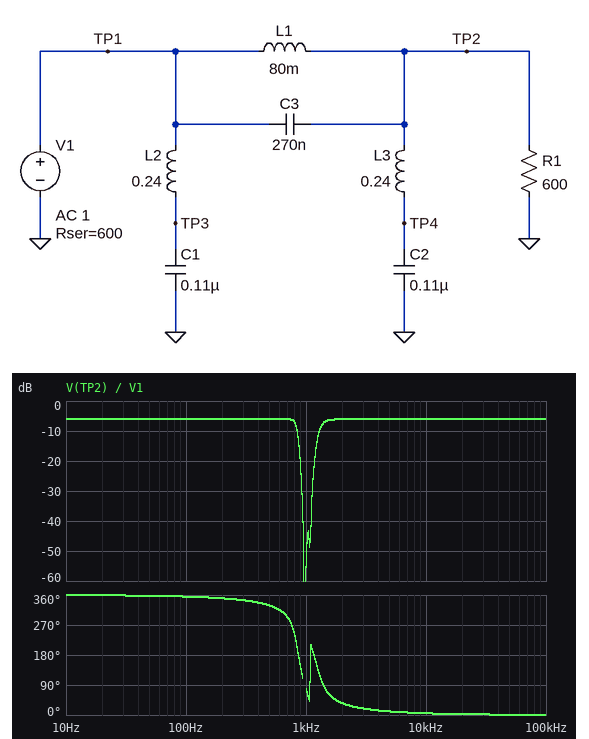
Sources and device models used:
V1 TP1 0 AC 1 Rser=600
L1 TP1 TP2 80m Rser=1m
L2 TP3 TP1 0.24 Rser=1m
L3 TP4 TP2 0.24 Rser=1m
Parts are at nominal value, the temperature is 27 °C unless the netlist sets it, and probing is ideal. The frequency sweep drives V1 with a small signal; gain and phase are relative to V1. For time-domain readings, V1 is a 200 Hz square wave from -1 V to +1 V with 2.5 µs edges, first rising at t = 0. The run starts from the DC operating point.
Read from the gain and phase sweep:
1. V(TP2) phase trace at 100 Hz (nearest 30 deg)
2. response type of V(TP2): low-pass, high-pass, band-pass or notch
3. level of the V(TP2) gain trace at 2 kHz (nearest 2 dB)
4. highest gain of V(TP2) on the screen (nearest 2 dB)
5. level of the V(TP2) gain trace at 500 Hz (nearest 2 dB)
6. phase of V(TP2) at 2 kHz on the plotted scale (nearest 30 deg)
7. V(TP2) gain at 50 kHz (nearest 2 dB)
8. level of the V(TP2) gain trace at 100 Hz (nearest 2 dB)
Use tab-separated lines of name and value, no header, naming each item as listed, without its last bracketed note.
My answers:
V(TP2) phase trace at 100 Hz	360 deg
response type of V(TP2): low-pass, high-pass, band-pass or notch	notch
level of the V(TP2) gain trace at 2 kHz	-6 dB
highest gain of V(TP2) on the screen	-6 dB
level of the V(TP2) gain trace at 500 Hz	-6 dB
phase of V(TP2) at 2 kHz on the plotted scale	30 deg
V(TP2) gain at 50 kHz	-6 dB
level of the V(TP2) gain trace at 100 Hz	-6 dB
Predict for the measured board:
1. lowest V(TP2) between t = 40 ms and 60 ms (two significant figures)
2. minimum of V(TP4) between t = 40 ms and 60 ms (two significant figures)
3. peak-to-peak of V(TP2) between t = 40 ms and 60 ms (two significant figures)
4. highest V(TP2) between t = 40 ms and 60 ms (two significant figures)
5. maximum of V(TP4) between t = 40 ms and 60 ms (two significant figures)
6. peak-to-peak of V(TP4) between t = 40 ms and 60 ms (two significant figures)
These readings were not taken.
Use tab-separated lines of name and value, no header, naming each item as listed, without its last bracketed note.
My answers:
lowest V(TP2) between t = 40 ms and 60 ms	-700 mV
minimum of V(TP4) between t = 40 ms and 60 ms	-730 mV
peak-to-peak of V(TP2) between t = 40 ms and 60 ms	1.4 V
highest V(TP2) between t = 40 ms and 60 ms	700 mV
maximum of V(TP4) between t = 40 ms and 60 ms	730 mV
peak-to-peak of V(TP4) between t = 40 ms and 60 ms	1.5 V
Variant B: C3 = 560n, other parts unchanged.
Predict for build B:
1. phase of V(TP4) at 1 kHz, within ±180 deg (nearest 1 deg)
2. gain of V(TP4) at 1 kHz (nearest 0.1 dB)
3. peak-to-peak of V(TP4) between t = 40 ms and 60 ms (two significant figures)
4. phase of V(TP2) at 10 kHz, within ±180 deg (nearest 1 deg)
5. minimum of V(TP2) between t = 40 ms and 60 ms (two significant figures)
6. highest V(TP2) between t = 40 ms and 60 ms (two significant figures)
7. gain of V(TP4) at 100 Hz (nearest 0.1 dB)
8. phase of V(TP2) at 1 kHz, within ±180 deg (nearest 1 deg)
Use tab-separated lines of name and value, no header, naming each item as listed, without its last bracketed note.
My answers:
phase of V(TP4) at 1 kHz, within ±180 deg	77 deg
gain of V(TP4) at 1 kHz	-11.3 dB
peak-to-peak of V(TP4) between t = 40 ms and 60 ms	1.7 V
phase of V(TP2) at 10 kHz, within ±180 deg	4 deg
minimum of V(TP2) between t = 40 ms and 60 ms	-720 mV
highest V(TP2) between t = 40 ms and 60 ms	720 mV
gain of V(TP4) at 100 Hz	-5.9 dB
phase of V(TP2) at 1 kHz, within ±180 deg	-103 deg
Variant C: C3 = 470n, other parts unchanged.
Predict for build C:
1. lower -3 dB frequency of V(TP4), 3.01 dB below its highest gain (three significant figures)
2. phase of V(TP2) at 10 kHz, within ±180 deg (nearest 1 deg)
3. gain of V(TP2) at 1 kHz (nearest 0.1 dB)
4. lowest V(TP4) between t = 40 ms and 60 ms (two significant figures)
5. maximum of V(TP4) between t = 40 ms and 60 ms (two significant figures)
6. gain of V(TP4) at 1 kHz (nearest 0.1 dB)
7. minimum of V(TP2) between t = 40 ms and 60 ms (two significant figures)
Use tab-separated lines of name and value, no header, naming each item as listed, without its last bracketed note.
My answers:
lower -3 dB frequency of V(TP4), 3.01 dB below its highest gain	1.06 kHz
phase of V(TP2) at 10 kHz, within ±180 deg	4 deg
gain of V(TP2) at 1 kHz	-43.5 dB
lowest V(TP4) between t = 40 ms and 60 ms	-780 mV
maximum of V(TP4) between t = 40 ms and 60 ms	780 mV
gain of V(TP4) at 1 kHz	-16.0 dB
minimum of V(TP2) between t = 40 ms and 60 ms	-720 mV
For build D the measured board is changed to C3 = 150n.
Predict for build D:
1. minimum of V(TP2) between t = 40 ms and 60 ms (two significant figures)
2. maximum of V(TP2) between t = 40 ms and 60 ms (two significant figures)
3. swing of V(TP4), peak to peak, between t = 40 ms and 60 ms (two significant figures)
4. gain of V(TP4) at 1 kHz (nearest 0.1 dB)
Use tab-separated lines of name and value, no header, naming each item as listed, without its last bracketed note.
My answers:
minimum of V(TP2) between t = 40 ms and 60 ms	-620 mV
maximum of V(TP2) between t = 40 ms and 60 ms	620 mV
swing of V(TP4), peak to peak, between t = 40 ms and 60 ms	1.6 V
gain of V(TP4) at 1 kHz	-17.4 dB
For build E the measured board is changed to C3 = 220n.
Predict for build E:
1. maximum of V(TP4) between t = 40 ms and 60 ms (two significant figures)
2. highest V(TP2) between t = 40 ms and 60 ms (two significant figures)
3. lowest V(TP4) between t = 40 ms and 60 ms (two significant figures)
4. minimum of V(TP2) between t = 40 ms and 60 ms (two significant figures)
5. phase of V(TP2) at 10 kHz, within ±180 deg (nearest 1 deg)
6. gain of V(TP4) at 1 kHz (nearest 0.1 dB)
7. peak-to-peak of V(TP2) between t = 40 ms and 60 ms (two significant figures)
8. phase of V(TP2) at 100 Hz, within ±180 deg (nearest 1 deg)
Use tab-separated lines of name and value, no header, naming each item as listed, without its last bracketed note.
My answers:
maximum of V(TP4) between t = 40 ms and 60 ms	750 mV
highest V(TP2) between t = 40 ms and 60 ms	670 mV
lowest V(TP4) between t = 40 ms and 60 ms	-750 mV
minimum of V(TP2) between t = 40 ms and 60 ms	-670 mV
phase of V(TP2) at 10 kHz, within ±180 deg	6 deg
gain of V(TP4) at 1 kHz	-21.7 dB
peak-to-peak of V(TP2) between t = 40 ms and 60 ms	1.3 V
phase of V(TP2) at 100 Hz, within ±180 deg	-5 deg
